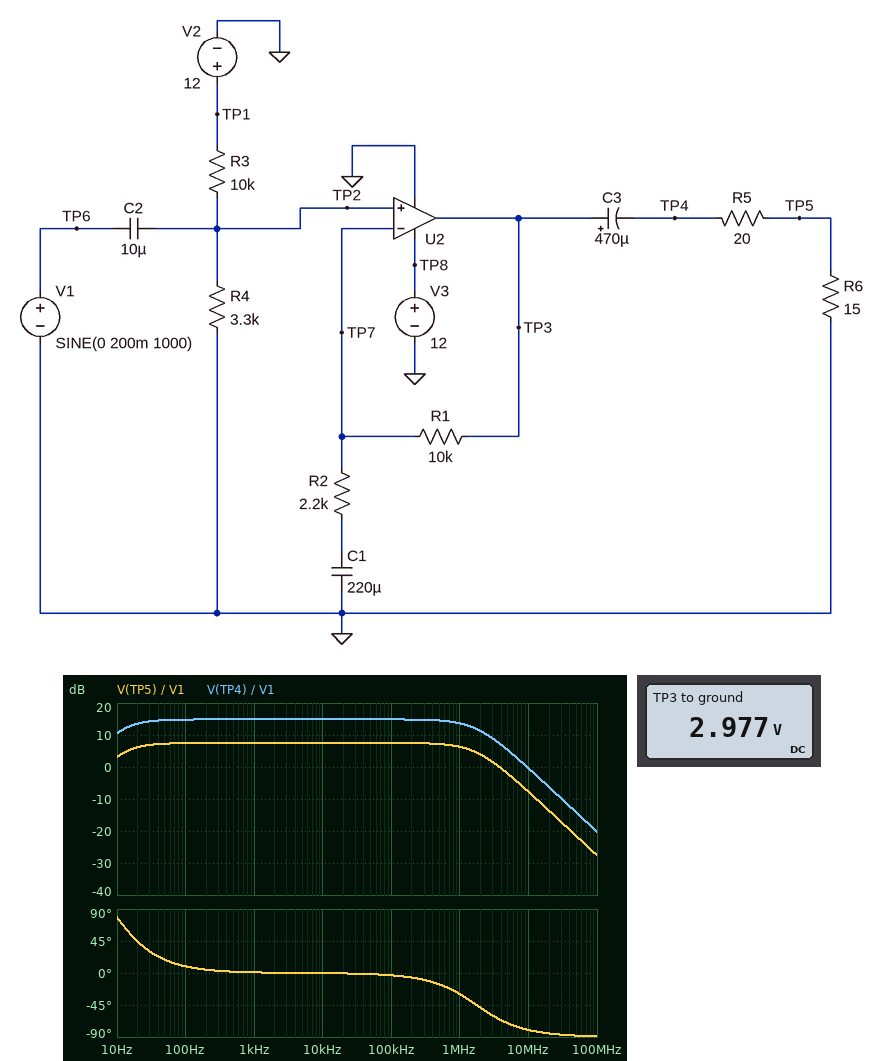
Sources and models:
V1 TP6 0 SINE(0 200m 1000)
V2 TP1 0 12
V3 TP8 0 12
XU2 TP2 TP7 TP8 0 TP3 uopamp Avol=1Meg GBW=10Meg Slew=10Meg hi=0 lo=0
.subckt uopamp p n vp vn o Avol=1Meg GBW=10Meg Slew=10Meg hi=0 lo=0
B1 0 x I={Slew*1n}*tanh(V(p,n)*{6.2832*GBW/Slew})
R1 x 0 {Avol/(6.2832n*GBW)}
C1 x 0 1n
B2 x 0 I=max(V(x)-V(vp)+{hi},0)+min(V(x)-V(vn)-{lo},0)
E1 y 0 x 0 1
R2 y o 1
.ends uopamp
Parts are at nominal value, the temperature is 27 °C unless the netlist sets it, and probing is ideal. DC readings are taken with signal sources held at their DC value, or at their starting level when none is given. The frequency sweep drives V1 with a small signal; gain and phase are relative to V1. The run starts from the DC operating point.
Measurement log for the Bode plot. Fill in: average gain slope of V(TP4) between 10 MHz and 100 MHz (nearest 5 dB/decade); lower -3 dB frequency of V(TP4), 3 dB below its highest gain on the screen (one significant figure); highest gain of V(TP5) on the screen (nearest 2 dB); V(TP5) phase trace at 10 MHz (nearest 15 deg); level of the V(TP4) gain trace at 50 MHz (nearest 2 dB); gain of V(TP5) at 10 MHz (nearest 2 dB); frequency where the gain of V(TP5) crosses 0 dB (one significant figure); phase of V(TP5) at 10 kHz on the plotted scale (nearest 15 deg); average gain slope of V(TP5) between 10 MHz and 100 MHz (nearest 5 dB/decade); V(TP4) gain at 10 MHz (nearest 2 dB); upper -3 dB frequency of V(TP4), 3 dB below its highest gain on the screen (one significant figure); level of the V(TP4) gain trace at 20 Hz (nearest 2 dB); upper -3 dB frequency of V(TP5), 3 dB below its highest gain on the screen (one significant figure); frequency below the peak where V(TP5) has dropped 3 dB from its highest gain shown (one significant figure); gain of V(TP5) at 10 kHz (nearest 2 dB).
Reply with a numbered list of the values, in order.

1. -20 dB/decade
2. 10 Hz
3. 8 dB
4. -75 deg
5. -14 dB
6. -8 dB
7. 4 MHz
8. 0 deg
9. -20 dB/decade
10. 0 dB
11. 2 MHz
12. 14 dB
13. 2 MHz
14. 10 Hz
15. 8 dB
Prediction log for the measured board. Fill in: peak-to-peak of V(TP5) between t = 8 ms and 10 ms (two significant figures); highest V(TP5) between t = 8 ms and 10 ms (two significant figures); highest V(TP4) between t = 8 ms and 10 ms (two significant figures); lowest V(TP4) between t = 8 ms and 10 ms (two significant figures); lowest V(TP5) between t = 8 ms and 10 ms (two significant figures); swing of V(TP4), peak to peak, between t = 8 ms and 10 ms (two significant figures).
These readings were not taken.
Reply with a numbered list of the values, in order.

1. 950 mV
2. 470 mV
3. 1.1 V
4. -1.1 V
5. -480 mV
6. 2.2 V
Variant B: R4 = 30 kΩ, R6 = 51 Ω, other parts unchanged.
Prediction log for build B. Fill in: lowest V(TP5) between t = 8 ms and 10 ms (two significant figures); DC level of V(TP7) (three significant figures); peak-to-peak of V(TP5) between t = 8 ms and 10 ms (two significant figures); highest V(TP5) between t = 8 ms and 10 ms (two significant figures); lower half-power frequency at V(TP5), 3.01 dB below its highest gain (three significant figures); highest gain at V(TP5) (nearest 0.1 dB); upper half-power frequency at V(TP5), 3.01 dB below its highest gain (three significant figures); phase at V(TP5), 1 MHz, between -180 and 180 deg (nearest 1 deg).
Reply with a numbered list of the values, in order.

1. -800 mV
2. 9.00 V
3. 1.6 V
4. 790 mV
5. 5.55 Hz
6. 12.0 dB
7. 1.78 MHz
8. -29 deg
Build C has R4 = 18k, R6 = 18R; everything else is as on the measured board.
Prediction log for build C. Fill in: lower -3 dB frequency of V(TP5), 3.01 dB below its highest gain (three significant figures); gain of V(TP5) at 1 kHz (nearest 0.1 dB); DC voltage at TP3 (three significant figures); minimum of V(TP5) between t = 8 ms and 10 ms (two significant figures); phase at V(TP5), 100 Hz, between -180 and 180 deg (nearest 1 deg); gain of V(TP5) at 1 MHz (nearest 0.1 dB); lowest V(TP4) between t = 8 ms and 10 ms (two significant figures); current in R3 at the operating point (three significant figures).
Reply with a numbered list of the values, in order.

1. 9.54 Hz
2. 8.4 dB
3. 7.71 V
4. -530 mV
5. 7 deg
6. 7.2 dB
7. -1.1 V
8. 429 µA
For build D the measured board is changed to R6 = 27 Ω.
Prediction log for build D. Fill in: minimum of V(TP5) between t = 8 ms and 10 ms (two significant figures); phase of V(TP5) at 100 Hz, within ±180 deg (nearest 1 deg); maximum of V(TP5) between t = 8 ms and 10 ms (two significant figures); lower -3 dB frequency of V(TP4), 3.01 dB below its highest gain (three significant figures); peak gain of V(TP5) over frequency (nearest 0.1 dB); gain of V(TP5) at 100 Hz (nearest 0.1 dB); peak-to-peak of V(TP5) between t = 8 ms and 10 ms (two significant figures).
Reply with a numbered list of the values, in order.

1. -640 mV
2. 8 deg
3. 630 mV
4. 10.6 Hz
5. 10.1 dB
6. 10.0 dB
7. 1.3 V
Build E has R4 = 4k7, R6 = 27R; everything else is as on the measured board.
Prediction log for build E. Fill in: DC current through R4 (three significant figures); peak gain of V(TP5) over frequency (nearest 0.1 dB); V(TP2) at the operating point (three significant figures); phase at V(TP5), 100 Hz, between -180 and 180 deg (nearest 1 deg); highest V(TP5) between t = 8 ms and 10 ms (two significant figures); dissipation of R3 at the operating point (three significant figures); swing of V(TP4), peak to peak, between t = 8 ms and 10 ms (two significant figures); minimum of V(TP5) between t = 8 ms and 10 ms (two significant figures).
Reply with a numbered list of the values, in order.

1. 816 µA
2. 10.1 dB
3. 3.84 V
4. 7 deg
5. 630 mV
6. 6.66 mW
7. 2.2 V
8. -640 mV
